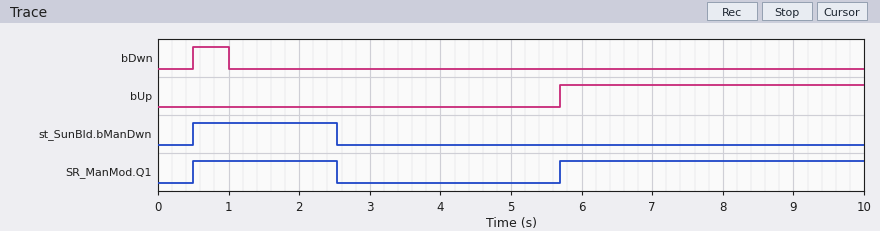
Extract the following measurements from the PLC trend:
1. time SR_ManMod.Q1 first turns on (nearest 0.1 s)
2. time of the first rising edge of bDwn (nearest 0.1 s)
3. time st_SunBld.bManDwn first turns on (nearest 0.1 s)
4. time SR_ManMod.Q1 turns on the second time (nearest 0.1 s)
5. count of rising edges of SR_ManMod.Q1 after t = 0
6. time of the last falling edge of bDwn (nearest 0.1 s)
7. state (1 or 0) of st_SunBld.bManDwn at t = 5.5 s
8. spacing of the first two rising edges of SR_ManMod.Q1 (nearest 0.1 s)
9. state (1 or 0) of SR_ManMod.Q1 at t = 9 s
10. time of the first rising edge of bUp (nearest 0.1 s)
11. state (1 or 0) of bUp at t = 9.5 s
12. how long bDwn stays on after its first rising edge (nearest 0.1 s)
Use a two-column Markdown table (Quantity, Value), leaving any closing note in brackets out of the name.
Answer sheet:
| Quantity | Value |
|---|---|
| time SR_ManMod.Q1 first turns on | 0.5 s |
| time of the first rising edge of bDwn | 0.5 s |
| time st_SunBld.bManDwn first turns on | 0.5 s |
| time SR_ManMod.Q1 turns on the second time | 5.7 s |
| count of rising edges of SR_ManMod.Q1 after t = 0 | 2 |
| time of the last falling edge of bDwn | 1.0 s |
| state (1 or 0) of st_SunBld.bManDwn at t = 5.5 s | 0 |
| spacing of the first two rising edges of SR_ManMod.Q1 | 5.2 s |
| state (1 or 0) of SR_ManMod.Q1 at t = 9 s | 1 |
| time of the first rising edge of bUp | 5.7 s |
| state (1 or 0) of bUp at t = 9.5 s | 1 |
| how long bDwn stays on after its first rising edge | 0.5 s |
